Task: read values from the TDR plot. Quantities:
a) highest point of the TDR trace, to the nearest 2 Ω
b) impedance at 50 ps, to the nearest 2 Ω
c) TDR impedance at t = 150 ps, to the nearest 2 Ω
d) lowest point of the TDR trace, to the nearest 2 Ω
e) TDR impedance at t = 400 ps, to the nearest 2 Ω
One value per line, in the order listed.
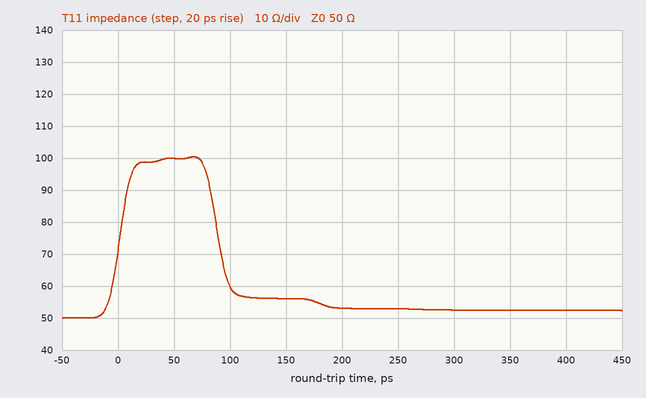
100 Ω
100 Ω
56 Ω
50 Ω
52 Ω
